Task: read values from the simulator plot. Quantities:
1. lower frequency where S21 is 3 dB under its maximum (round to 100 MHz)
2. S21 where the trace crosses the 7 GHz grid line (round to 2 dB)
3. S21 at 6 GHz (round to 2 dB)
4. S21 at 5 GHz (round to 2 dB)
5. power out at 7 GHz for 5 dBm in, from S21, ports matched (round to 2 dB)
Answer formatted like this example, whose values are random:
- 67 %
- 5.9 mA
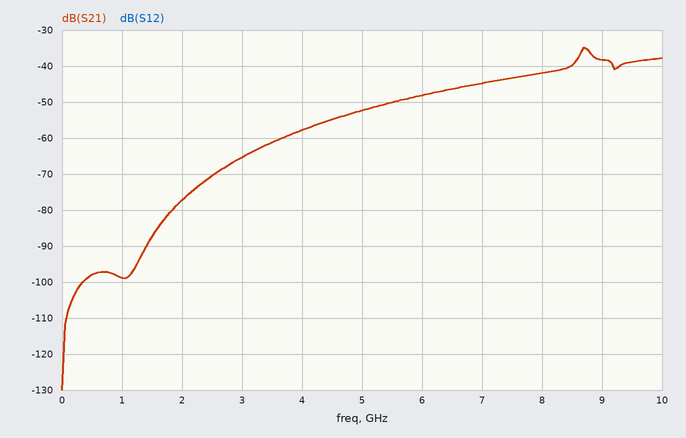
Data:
- 8.6 GHz
- -44 dB
- -48 dB
- -52 dB
- -40 dBm
